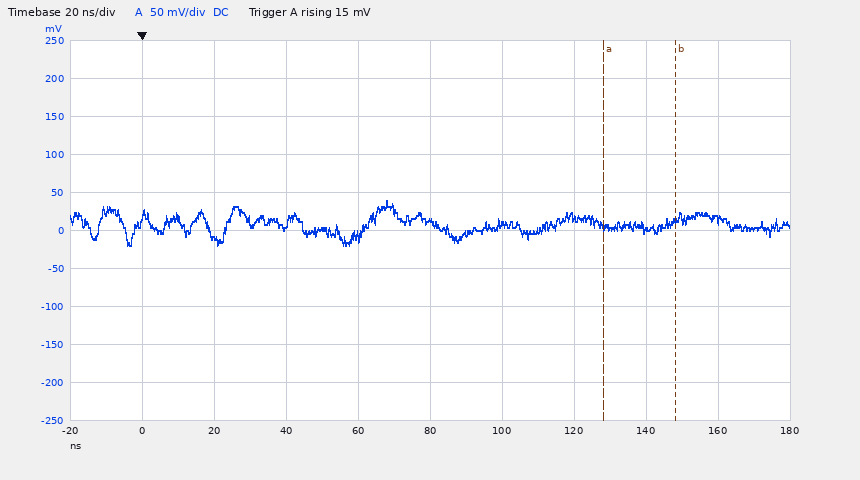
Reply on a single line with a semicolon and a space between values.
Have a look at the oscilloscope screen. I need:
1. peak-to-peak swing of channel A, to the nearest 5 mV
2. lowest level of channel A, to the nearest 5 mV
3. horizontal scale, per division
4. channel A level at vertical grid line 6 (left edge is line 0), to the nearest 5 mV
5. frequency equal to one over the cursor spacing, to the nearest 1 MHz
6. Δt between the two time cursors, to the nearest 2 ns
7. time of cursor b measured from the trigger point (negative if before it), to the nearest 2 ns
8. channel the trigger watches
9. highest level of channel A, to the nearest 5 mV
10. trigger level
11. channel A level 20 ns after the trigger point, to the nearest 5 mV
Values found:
60 mV; -20 mV; 20 ns; 10 mV; 50 MHz; 20 ns; +148 ns; channel A; 40 mV; 15 mV; -10 mV
